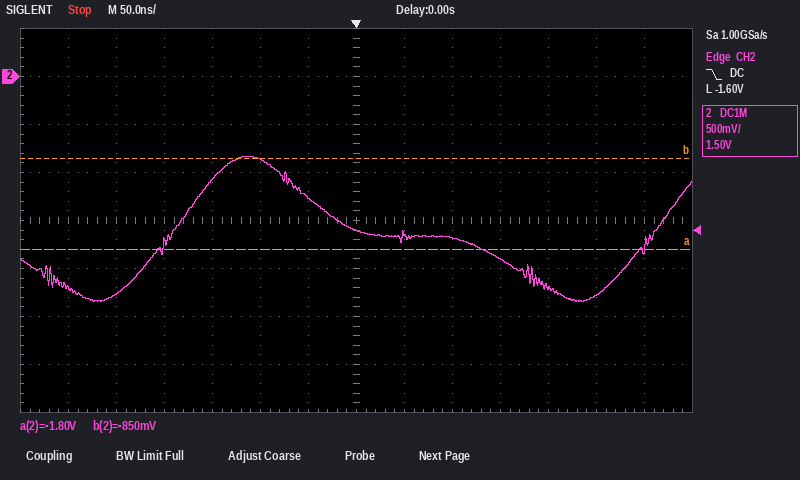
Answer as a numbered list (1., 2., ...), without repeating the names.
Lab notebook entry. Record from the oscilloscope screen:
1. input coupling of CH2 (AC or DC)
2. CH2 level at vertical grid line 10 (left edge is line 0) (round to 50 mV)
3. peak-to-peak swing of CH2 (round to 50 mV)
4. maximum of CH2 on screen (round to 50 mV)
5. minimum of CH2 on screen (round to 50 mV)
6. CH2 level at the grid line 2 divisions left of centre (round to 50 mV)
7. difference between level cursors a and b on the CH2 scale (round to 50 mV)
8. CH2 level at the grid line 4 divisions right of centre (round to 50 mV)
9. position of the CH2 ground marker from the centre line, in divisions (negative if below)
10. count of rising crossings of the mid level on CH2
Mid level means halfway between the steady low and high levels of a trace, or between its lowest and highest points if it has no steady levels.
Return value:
1. DC
2. -1.90 V
3. 1.50 V
4. -850 mV
5. -2.35 V
6. -850 mV
7. 950 mV
8. -2.20 V
9. +3.0 div
10. 2
